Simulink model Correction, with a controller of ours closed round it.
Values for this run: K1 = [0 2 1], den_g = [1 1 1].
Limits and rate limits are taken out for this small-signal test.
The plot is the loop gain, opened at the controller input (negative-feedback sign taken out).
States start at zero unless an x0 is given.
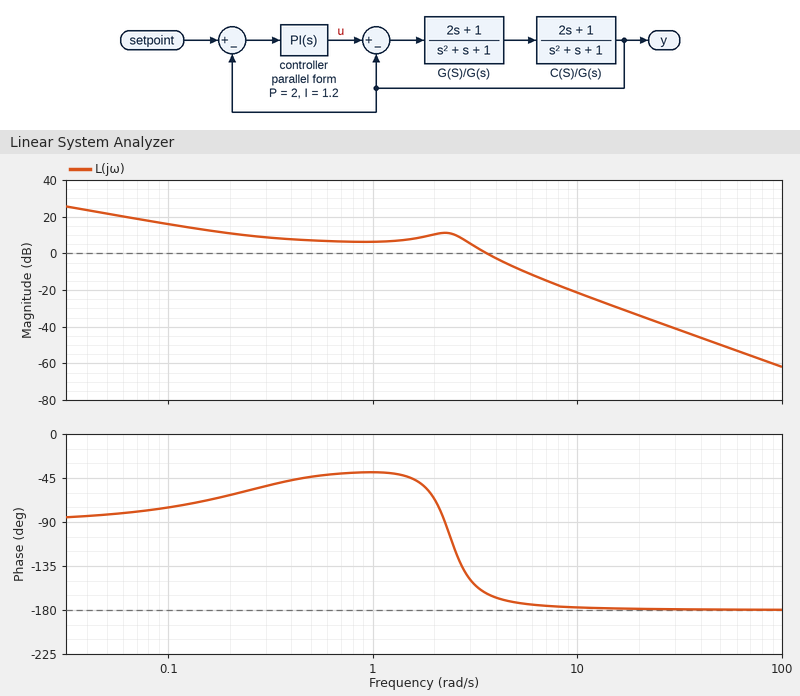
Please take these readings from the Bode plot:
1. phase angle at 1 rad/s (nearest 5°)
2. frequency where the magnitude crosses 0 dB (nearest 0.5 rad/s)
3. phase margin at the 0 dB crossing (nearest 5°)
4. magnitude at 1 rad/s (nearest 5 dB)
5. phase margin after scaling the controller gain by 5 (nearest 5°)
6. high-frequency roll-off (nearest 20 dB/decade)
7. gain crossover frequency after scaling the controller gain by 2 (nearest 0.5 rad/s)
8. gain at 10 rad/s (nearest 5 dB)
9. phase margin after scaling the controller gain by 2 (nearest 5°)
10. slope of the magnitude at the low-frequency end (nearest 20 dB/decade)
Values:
-40°
3.5 rad/s
15°
5 dB
5°
-40 dB/decade
4.5 rad/s
-20 dB
10°
-20 dB/decade
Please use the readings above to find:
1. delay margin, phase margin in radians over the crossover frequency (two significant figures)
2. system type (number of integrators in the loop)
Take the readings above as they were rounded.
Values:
0.075 s
1
